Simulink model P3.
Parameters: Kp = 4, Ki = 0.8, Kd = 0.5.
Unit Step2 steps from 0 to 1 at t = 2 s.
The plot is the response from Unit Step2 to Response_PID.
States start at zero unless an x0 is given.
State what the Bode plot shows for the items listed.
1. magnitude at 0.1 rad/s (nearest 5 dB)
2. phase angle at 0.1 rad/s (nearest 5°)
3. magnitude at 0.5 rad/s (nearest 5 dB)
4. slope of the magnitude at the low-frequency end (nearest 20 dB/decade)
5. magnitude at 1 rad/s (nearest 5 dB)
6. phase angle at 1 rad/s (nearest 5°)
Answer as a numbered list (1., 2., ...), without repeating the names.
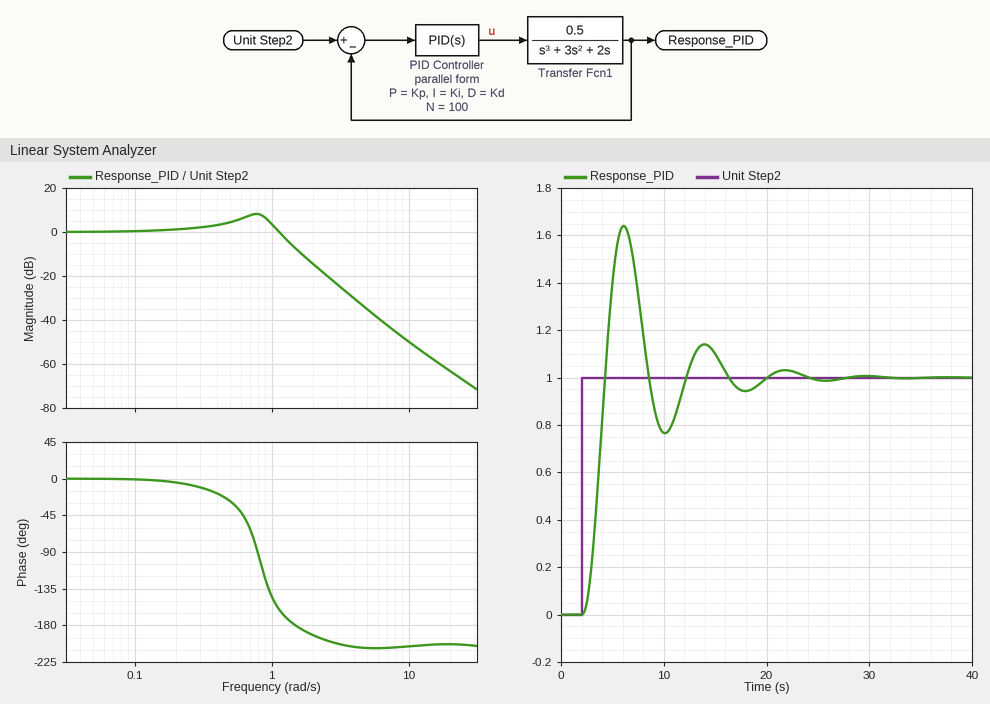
1. 0 dB
2. 0°
3. 5 dB
4. 0 dB/decade
5. 5 dB
6. -145°
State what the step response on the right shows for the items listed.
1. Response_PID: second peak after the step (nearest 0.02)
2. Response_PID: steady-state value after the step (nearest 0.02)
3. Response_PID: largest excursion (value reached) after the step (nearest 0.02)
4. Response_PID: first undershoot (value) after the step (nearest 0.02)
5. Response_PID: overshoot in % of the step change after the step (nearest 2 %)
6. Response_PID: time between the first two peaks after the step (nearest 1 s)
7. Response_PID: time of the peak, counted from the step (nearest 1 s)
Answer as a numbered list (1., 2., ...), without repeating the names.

1. 1.14
2. 1.00
3. 1.64
4. 0.76
5. 64 %
6. 8 s
7. 4 s
